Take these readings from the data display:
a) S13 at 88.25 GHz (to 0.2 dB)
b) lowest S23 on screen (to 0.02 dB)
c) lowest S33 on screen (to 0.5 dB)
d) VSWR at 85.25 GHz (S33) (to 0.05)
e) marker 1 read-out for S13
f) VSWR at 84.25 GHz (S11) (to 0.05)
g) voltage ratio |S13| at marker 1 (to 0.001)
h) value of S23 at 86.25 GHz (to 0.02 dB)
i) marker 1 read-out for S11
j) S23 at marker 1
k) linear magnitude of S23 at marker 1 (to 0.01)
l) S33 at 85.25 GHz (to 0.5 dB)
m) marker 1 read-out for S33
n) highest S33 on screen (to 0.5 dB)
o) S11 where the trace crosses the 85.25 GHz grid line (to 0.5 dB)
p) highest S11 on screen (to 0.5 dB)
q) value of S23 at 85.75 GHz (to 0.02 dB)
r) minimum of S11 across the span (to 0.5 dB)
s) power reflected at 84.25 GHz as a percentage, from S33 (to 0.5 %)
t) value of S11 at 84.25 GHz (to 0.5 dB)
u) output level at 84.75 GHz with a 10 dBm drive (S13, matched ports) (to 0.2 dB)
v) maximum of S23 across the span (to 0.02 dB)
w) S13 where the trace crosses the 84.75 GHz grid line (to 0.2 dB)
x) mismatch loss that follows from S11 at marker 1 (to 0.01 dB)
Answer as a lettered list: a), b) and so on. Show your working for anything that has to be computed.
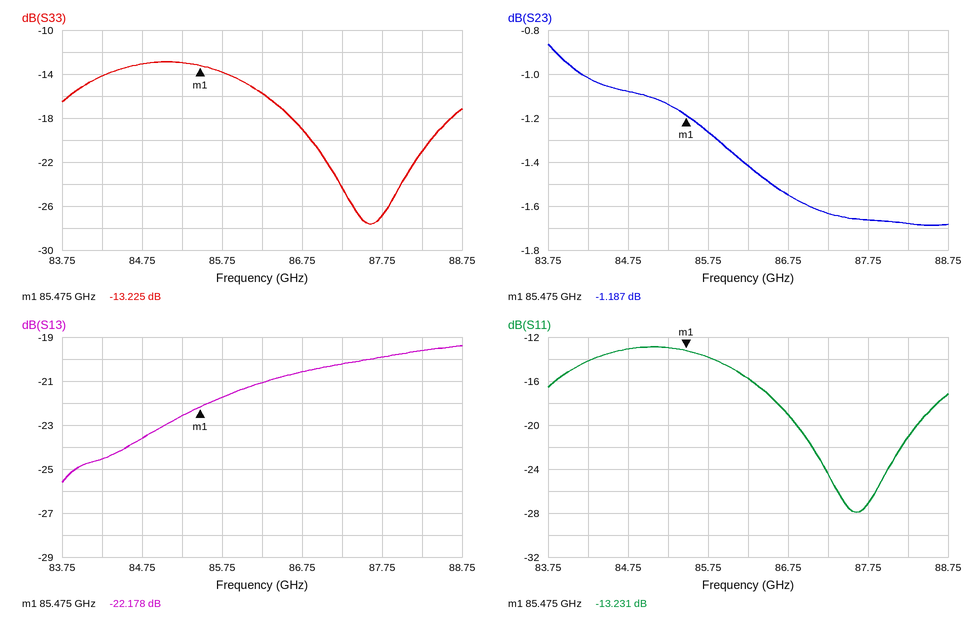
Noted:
a) -19.6 dB
b) -1.68 dB
c) -27.5 dB
d) |Γ| = 10^(-13/20) = 0.2239; VSWR = (1 + 0.2239)/(1 − 0.2239) ≈ 1.58, so 1.60 to the nearest 0.05
e) -22.178 dB
f) |Γ| = 10^(-14/20) = 0.1995; VSWR = (1 + 0.1995)/(1 − 0.1995) ≈ 1.50
g) 10^(-22.178/20) ≈ 0.078
h) -1.42 dB
i) -13.231 dB
j) -1.187 dB
k) 10^(-1.187/20) ≈ 0.87
l) -13.0 dB
m) -13.225 dB
n) -13.0 dB
o) -13.0 dB
p) -13.0 dB
q) -1.26 dB
r) -28.0 dB
s) 10^(-14/10) ≈ 4.0 %
t) -14.0 dB
u) 10 dBm + (-23.6 dB) = -13.6 dBm
v) -0.86 dB
w) -23.6 dB
x) −10 log10(1 − 10^(-13.231/10)) ≈ 0.21 dB
